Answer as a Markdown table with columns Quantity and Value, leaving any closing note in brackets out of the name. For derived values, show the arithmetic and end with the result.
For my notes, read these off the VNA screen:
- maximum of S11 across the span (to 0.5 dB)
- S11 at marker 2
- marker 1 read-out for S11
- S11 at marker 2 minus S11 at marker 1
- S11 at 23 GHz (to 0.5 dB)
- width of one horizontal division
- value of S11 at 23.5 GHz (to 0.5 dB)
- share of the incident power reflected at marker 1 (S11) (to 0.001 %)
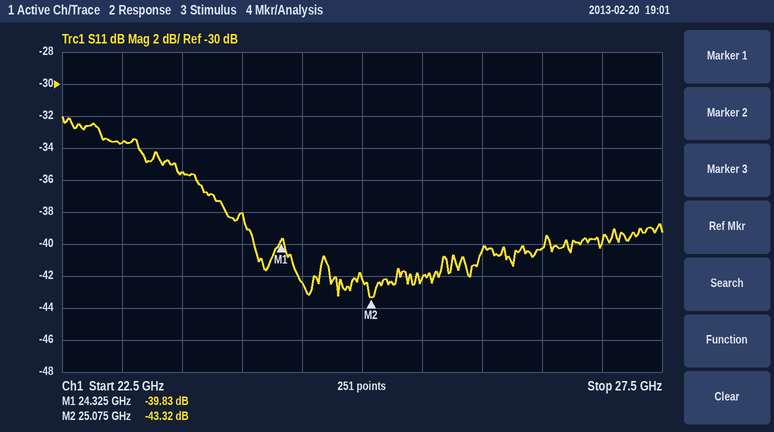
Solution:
| Quantity | Value |
|---|---|
| maximum of S11 across the span | -32.0 dB |
| S11 at marker 2 | -43.32 dB |
| marker 1 read-out for S11 | -39.83 dB |
| S11 at marker 2 minus S11 at marker 1 | -43.32 − (-39.83) = -3.49 dB |
| S11 at 23 GHz | -33.5 dB |
| width of one horizontal division | 500 MHz |
| value of S11 at 23.5 GHz | -35.5 dB |
| share of the incident power reflected at marker 1 (S11) | 10^(-39.83/10) ≈ 0.010 % |
